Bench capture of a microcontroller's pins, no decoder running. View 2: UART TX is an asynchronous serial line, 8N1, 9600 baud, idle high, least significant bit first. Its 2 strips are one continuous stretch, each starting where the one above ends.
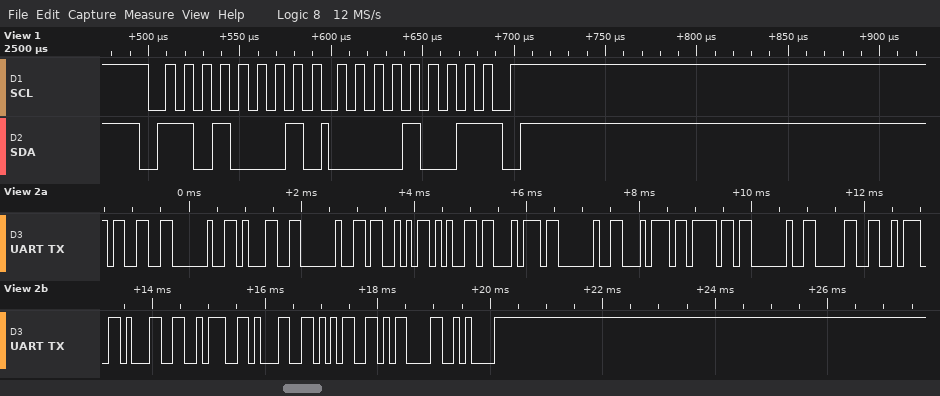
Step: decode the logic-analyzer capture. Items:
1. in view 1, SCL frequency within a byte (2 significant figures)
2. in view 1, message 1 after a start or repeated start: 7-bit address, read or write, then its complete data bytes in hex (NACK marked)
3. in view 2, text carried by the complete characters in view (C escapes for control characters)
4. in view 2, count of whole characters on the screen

100 kHz
0x68 read: 09 NACK
"3 1 Set to 0:1:15\r\n"
19
